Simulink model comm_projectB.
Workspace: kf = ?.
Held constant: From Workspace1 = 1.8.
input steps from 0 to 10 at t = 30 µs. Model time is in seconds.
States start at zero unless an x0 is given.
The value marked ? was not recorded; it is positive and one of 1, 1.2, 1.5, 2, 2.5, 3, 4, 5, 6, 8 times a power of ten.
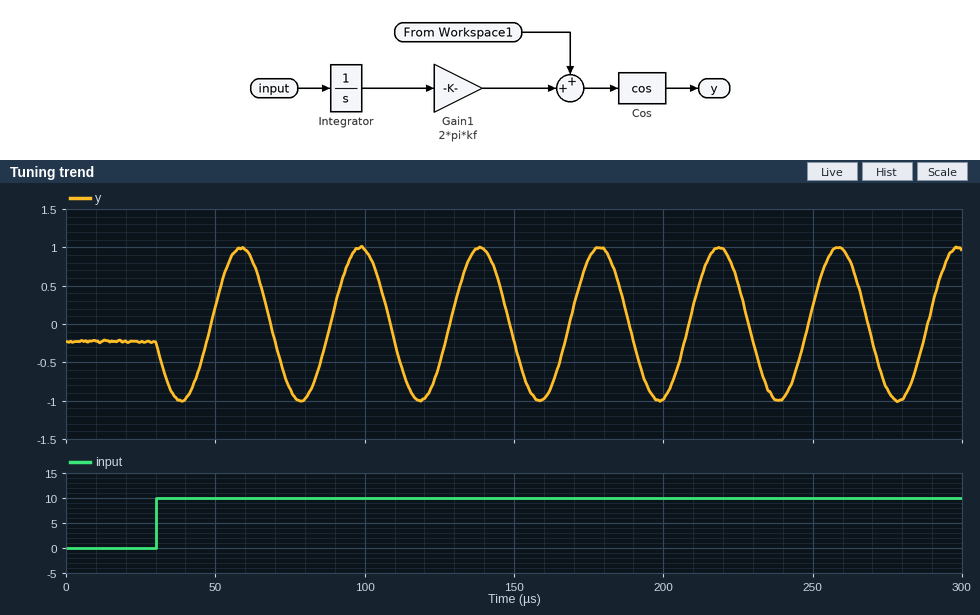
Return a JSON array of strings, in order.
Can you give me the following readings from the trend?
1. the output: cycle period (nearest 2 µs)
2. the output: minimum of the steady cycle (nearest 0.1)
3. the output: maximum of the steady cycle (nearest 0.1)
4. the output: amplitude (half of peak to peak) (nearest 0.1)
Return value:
["40 µs", "-1.0", "1.0", "1.0"]
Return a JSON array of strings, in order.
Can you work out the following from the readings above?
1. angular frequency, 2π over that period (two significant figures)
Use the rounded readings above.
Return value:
["0.16 rad/µs"]
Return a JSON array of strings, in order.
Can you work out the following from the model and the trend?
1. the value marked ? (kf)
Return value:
["2500"]
